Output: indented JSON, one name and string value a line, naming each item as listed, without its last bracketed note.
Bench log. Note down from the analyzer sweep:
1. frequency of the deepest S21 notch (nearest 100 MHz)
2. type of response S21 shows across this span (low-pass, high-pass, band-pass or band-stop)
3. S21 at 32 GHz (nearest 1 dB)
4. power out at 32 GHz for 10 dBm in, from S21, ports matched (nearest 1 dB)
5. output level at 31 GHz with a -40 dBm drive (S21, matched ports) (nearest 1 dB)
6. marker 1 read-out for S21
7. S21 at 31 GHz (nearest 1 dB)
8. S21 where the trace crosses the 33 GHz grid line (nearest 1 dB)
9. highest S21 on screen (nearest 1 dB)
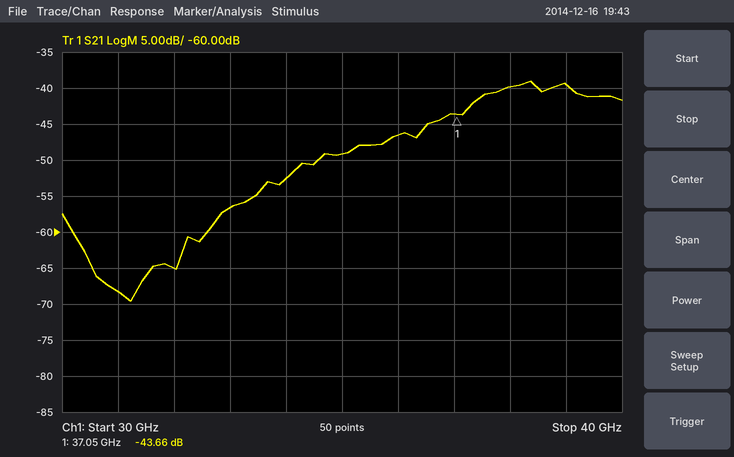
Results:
{
  "frequency of the deepest S21 notch": "31.2 GHz",
  "type of response S21 shows across this span": "high-pass",
  "S21 at 32 GHz": "-65 dB",
  "power out at 32 GHz for 10 dBm in, from S21, ports matched": "-55 dBm",
  "output level at 31 GHz with a -40 dBm drive (S21, matched ports)": "-108 dBm",
  "marker 1 read-out for S21": "-43.66 dB",
  "S21 at 31 GHz": "-68 dB",
  "S21 where the trace crosses the 33 GHz grid line": "-57 dB",
  "highest S21 on screen": "-39 dB"
}
